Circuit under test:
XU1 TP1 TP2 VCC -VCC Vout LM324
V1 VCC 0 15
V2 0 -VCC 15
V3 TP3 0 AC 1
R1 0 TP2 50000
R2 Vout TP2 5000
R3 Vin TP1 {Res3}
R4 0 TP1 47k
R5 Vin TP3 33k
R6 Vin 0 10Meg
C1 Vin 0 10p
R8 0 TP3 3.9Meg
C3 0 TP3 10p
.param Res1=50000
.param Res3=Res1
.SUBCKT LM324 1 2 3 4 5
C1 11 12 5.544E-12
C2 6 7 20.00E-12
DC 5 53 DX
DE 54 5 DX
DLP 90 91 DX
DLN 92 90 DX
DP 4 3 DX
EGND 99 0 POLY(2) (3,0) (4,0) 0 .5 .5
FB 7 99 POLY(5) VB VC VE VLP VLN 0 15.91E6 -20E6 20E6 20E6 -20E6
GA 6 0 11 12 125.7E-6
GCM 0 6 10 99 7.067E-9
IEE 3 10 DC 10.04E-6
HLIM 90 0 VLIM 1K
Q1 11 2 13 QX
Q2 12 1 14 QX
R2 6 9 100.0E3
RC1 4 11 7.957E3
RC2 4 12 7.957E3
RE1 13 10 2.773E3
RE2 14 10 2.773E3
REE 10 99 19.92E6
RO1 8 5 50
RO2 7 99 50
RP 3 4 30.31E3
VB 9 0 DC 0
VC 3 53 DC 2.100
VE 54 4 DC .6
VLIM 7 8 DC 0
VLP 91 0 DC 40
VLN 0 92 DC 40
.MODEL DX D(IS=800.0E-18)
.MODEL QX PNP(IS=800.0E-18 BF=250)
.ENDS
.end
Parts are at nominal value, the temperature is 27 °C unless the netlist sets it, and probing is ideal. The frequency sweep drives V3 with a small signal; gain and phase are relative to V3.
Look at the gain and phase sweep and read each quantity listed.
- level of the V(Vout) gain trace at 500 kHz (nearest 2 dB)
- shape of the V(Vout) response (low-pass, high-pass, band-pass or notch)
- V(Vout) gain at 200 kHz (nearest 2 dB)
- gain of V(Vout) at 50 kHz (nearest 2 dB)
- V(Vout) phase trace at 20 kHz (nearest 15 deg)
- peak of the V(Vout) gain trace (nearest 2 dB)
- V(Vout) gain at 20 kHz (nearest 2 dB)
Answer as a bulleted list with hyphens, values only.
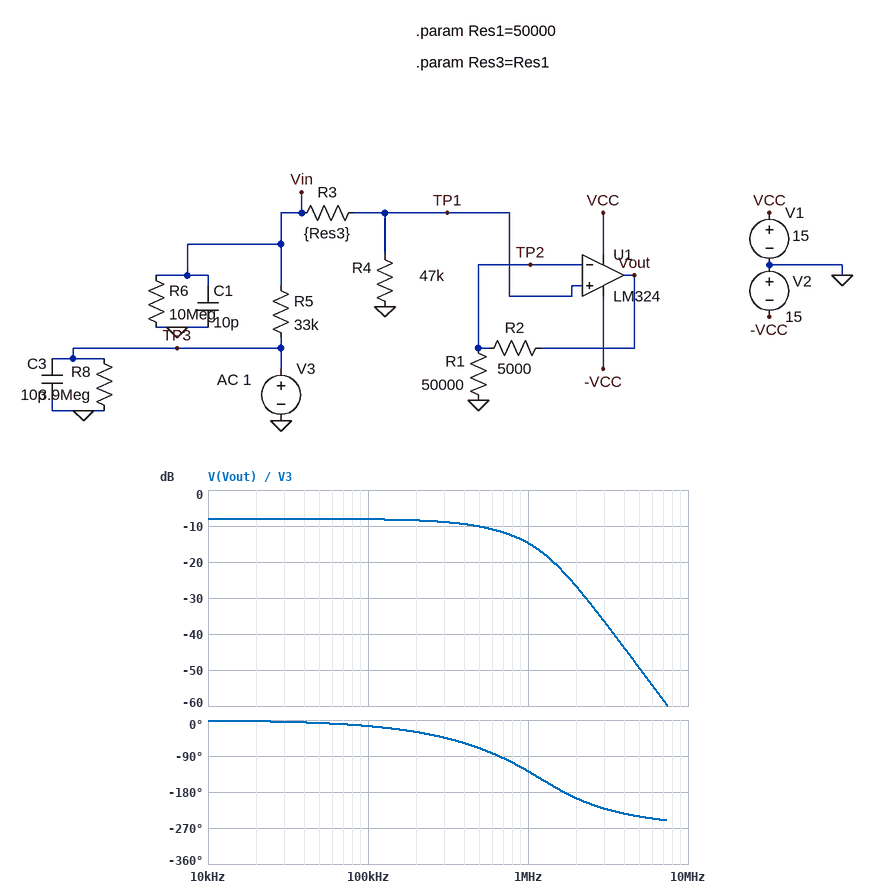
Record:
- -10 dB
- low-pass
- -8 dB
- -8 dB
- 0 deg
- -8 dB
- -8 dB
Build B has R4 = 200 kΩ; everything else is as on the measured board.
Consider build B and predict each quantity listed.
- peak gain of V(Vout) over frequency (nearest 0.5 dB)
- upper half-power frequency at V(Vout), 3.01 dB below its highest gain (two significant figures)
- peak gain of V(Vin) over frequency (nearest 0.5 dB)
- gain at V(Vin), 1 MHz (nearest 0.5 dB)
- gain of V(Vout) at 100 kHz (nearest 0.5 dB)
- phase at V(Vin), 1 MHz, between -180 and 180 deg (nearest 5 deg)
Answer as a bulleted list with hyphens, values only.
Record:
- -2.0 dB
- 530 kHz
- -1.0 dB
- -7.5 dB
- -2.5 dB
- -60 deg
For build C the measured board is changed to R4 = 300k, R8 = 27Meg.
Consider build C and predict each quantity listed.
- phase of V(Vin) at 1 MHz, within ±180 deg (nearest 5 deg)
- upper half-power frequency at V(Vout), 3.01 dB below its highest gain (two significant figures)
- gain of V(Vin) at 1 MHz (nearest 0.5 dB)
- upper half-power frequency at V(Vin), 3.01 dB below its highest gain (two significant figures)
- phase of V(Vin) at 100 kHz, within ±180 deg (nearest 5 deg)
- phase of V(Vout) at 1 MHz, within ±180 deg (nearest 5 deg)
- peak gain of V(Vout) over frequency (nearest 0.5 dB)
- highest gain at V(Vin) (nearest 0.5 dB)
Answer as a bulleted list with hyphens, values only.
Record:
- -60 deg
- 510 kHz
- -7.5 dB
- 530 kHz
- -10 deg
- -135 deg
- -1.5 dB
- -1.0 dB
